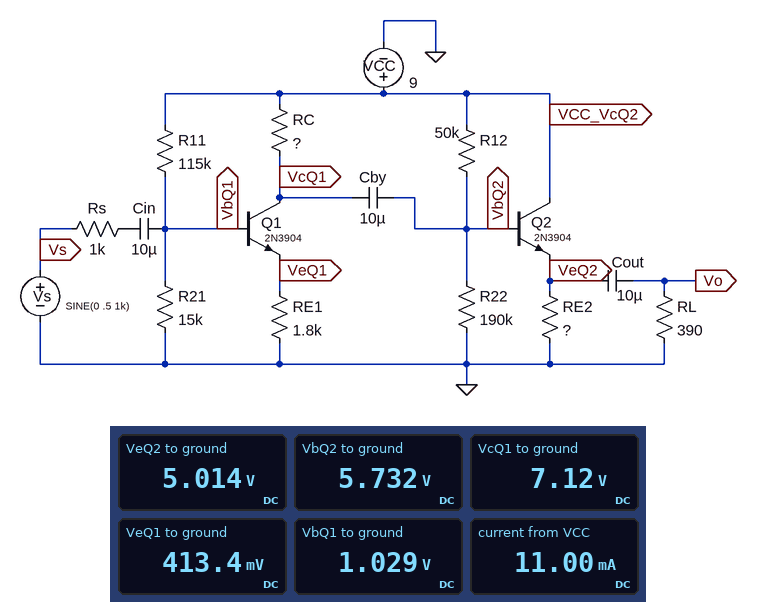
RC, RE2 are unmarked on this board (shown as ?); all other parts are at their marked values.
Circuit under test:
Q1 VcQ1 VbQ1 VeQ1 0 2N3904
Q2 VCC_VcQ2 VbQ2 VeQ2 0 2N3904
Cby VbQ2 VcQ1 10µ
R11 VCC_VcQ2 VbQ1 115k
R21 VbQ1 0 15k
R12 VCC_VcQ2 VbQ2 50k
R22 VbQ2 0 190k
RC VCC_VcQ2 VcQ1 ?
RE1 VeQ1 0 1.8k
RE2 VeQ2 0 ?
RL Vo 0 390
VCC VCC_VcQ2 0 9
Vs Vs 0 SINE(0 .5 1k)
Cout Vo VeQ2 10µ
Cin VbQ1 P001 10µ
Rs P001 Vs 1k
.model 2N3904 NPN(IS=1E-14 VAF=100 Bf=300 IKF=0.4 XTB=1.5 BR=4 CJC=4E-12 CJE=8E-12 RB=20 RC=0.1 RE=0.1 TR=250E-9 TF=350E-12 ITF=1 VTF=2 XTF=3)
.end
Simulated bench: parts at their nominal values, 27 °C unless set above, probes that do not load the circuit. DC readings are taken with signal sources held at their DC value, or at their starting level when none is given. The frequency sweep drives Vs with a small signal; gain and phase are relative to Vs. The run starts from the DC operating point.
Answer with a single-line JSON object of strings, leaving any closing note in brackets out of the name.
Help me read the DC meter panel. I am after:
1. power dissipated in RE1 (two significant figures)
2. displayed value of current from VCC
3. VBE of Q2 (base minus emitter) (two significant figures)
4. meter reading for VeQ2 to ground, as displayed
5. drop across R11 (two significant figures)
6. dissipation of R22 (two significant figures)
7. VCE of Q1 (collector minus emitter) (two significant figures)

{"power dissipated in RE1": "95 µW", "displayed value of current from VCC": "11.00 mA", "VBE of Q2 (base minus emitter)": "720 mV", "meter reading for VeQ2 to ground, as displayed": "5.014 V", "drop across R11": "8.0 V", "dissipation of R22": "170 µW", "VCE of Q1 (collector minus emitter)": "6.7 V"}
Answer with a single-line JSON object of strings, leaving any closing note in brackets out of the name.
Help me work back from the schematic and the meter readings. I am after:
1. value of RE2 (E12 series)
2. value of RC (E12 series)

{"value of RE2": "470 Ω", "value of RC": "8.2 kΩ"}
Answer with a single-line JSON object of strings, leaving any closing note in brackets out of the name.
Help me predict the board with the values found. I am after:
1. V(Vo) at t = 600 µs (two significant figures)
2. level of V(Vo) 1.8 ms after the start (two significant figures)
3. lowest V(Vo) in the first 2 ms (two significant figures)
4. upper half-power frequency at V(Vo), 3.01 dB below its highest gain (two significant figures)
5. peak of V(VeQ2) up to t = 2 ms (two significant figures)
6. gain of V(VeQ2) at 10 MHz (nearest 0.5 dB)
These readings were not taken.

{"V(Vo) at t = 600 µs": "930 mV", "level of V(Vo) 1.8 ms after the start": "1.3 V", "lowest V(Vo) in the first 2 ms": "-1.4 V", "upper half-power frequency at V(Vo), 3.01 dB below its highest gain": "3.7 MHz", "peak of V(VeQ2) up to t = 2 ms": "6.3 V", "gain of V(VeQ2) at 10 MHz": "0.5 dB"}
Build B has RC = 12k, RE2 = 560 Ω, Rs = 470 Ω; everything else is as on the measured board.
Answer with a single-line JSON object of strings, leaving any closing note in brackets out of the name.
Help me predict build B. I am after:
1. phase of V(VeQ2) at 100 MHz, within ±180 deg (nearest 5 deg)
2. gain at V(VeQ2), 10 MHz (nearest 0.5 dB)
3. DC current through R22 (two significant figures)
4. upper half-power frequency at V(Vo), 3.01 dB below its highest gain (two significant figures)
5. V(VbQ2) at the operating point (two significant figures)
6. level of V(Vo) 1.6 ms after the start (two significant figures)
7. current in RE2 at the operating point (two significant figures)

{"phase of V(VeQ2) at 100 MHz, within ±180 deg": "-10 deg", "gain at V(VeQ2), 10 MHz": "1.5 dB", "DC current through R22": "31 µA", "upper half-power frequency at V(Vo), 3.01 dB below its highest gain": "3.0 MHz", "V(VbQ2) at the operating point": "5.9 V", "level of V(Vo) 1.6 ms after the start": "1.3 V", "current in RE2 at the operating point": "9.3 mA"}
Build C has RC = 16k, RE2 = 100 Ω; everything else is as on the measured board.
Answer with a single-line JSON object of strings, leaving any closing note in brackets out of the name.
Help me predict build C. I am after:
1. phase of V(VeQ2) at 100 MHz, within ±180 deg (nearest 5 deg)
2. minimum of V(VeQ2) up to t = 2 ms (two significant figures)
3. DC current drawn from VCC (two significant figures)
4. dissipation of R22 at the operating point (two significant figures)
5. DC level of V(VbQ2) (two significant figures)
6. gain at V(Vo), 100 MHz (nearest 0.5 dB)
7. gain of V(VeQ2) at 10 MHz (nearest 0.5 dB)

{"phase of V(VeQ2) at 100 MHz, within ±180 deg": "-25 deg", "minimum of V(VeQ2) up to t = 2 ms": "890 mV", "DC current drawn from VCC": "28 mA", "dissipation of R22 at the operating point": "64 µW", "DC level of V(VbQ2)": "3.5 V", "gain at V(Vo), 100 MHz": "-16.5 dB", "gain of V(VeQ2) at 10 MHz": "-2.0 dB"}
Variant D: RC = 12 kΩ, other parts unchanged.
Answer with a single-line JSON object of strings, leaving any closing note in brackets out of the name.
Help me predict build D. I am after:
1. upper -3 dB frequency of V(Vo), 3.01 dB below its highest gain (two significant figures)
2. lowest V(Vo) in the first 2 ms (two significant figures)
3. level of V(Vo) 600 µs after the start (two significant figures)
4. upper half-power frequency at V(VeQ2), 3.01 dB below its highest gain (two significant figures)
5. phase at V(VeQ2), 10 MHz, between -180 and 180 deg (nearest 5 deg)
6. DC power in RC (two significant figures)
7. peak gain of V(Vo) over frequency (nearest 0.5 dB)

{"upper -3 dB frequency of V(Vo), 3.01 dB below its highest gain": "2.8 MHz", "lowest V(Vo) in the first 2 ms": "-1.9 V", "level of V(Vo) 600 µs after the start": "1.2 V", "upper half-power frequency at V(VeQ2), 3.01 dB below its highest gain": "2.4 MHz", "phase at V(VeQ2), 10 MHz, between -180 and 180 deg": "80 deg", "DC power in RC": "630 µW", "peak gain of V(Vo) over frequency": "11.5 dB"}
